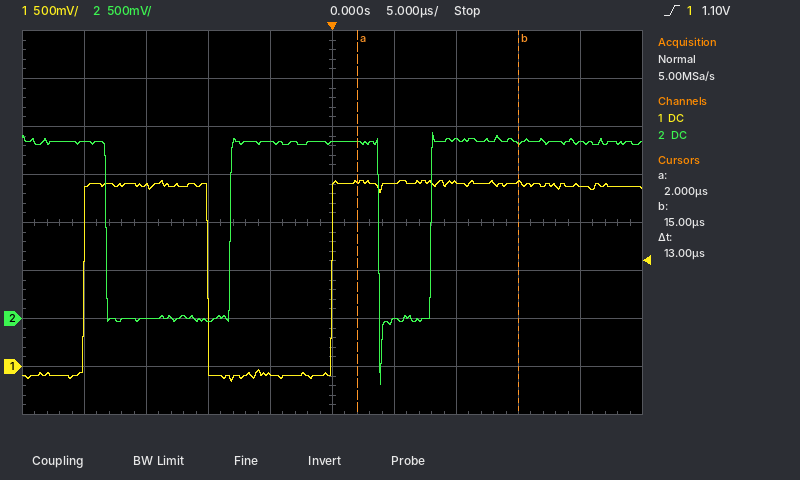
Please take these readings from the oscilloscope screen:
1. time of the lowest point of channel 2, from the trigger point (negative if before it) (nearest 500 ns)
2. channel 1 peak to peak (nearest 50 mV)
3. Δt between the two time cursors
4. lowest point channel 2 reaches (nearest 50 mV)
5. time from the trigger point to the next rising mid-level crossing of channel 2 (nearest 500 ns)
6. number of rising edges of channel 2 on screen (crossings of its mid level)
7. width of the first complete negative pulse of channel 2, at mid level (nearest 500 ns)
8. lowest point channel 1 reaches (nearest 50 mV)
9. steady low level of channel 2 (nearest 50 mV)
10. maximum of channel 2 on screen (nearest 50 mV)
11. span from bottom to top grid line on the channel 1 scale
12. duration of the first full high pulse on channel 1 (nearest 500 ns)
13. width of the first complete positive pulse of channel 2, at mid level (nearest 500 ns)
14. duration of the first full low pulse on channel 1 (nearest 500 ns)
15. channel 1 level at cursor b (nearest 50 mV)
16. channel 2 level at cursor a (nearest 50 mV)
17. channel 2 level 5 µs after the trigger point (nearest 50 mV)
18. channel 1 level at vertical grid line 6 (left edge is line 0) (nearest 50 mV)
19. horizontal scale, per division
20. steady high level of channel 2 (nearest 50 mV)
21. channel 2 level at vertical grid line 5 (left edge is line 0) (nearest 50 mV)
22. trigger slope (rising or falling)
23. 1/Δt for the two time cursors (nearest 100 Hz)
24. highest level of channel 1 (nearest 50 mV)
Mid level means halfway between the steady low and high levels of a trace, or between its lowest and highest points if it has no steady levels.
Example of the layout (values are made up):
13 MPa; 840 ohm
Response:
+4.0 µs; 2.10 V; 13 µs; -700 mV; 8.0 µs; 2; 10.0 µs; -150 mV; 0 mV; 1.95 V; 4 V; 10.0 µs; 12.0 µs; 10.0 µs; 1.90 V; 1.85 V; 0 mV; 1.90 V; 5 µs; 1.85 V; 1.85 V; rising; 76.9 kHz; 1.95 V
